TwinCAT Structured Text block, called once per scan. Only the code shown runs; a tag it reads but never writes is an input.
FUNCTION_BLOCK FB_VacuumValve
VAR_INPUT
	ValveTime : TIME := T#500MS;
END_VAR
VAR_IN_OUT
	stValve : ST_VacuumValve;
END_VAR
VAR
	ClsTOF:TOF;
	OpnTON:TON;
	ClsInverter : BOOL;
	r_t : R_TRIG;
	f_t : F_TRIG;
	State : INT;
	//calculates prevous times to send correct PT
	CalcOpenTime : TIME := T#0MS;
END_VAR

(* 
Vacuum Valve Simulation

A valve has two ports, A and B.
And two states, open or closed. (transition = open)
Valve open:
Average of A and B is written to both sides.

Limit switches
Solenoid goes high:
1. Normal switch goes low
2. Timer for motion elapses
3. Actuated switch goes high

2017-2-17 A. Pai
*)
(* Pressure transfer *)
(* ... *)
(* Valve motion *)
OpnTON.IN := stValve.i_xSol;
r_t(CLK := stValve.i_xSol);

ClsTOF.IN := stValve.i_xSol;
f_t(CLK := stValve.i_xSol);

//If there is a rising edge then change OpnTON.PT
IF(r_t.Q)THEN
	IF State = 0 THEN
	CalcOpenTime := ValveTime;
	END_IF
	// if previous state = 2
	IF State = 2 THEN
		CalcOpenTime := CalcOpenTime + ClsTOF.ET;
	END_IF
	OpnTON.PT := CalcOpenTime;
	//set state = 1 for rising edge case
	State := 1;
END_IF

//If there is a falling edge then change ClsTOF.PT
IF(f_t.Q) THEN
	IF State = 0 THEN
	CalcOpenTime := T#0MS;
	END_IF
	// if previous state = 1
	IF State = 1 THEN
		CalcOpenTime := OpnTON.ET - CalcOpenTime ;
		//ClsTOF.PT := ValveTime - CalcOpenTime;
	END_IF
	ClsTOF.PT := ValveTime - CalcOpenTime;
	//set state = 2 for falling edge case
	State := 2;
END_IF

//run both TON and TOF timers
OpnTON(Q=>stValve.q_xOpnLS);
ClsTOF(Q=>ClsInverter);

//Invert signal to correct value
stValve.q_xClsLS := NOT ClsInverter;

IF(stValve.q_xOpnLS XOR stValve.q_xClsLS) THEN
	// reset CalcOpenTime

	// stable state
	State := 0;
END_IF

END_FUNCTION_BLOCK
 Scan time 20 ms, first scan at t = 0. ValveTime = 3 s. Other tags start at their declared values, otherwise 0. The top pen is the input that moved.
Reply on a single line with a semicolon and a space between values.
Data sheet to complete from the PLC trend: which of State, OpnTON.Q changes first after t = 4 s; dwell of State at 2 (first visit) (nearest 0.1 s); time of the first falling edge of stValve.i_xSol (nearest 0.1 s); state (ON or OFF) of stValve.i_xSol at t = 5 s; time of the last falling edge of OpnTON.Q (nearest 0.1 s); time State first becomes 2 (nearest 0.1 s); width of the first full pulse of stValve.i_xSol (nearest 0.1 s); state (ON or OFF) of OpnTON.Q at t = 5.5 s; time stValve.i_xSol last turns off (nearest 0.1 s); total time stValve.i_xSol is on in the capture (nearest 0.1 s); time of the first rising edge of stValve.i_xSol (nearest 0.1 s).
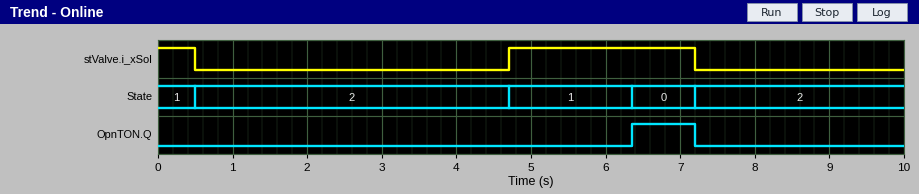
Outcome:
State; 4.2 s; 0.5 s; ON; 7.2 s; 0.5 s; 2.5 s; OFF; 7.2 s; 3.0 s; 4.7 s
